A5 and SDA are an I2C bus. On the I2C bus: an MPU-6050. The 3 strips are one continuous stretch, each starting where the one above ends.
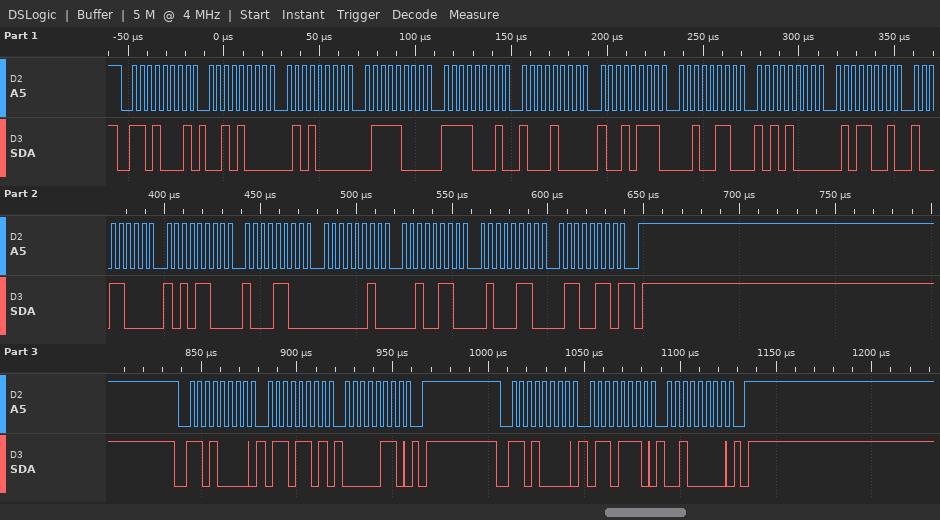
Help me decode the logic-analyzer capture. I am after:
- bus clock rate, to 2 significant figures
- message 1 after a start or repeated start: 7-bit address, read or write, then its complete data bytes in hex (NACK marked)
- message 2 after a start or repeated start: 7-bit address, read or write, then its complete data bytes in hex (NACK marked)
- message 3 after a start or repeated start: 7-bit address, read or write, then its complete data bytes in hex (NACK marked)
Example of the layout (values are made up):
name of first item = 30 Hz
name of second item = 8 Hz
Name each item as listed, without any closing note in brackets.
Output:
bus clock rate, to 2 significant figures = 250 kHz
message 1 after a start or repeated start: 7-bit address, read or write, then its complete data bytes in hex = 0x68 read: 28 50 78 F1 88 97 26 A8 59 98 AC 8C 02 26 46 66 NACK
message 2 after a start or repeated start: 7-bit address, read or write, then its complete data bytes in hex = 0x68 write: 6D 06
message 3 after a start or repeated start: 7-bit address, read or write, then its complete data bytes in hex = 0x68 write: 6E 20
